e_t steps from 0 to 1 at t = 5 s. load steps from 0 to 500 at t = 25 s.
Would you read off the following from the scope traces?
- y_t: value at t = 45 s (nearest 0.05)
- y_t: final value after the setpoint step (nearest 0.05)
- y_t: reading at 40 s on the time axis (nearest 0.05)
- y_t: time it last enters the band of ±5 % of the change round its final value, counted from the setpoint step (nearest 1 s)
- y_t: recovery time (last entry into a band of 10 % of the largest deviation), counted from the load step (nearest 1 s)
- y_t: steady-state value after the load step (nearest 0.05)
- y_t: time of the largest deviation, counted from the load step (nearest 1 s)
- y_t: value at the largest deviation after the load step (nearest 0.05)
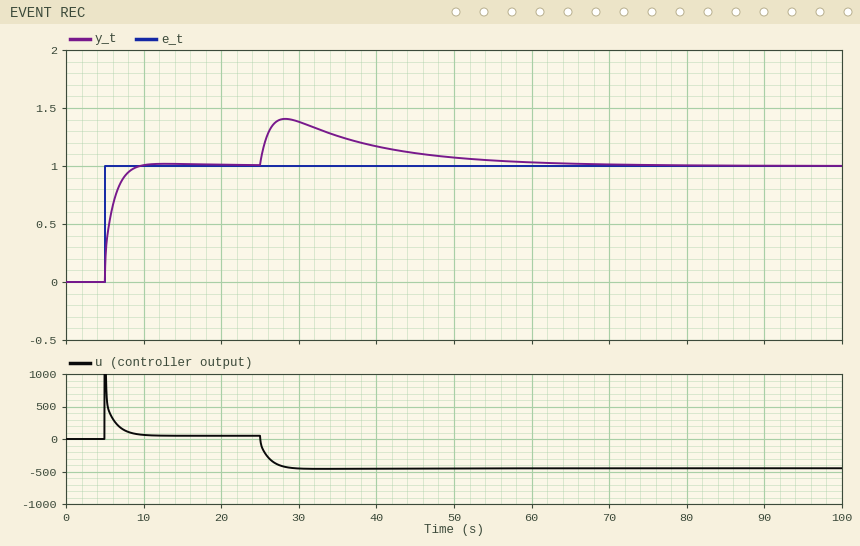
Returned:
1.10
1.00
1.15
3 s
32 s
1.00
3 s
1.40
